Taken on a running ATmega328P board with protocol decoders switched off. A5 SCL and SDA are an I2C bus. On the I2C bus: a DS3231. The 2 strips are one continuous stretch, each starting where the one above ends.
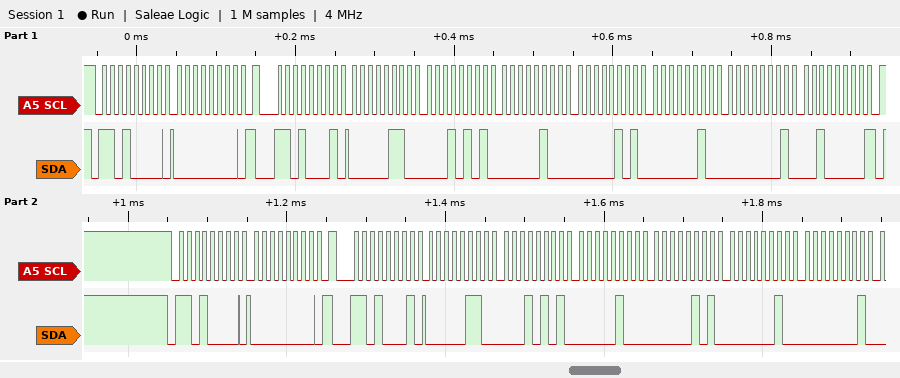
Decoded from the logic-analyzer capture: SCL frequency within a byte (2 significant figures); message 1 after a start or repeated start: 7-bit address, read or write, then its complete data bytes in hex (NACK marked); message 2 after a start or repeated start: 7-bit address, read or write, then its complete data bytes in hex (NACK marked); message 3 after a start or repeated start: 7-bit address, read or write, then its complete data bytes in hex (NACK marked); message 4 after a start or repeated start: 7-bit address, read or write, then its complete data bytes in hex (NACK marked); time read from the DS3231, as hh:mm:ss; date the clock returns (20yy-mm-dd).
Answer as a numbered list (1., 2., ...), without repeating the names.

1. 100 kHz
2. 0x68 write: 00
3. 0x68 read: 06 15 04 05 02 01 20 NACK
4. 0x68 write: 00
5. 0x68 read: 06 15 04 05 02 01
6. 04:15:06
7. 2020-01-02
